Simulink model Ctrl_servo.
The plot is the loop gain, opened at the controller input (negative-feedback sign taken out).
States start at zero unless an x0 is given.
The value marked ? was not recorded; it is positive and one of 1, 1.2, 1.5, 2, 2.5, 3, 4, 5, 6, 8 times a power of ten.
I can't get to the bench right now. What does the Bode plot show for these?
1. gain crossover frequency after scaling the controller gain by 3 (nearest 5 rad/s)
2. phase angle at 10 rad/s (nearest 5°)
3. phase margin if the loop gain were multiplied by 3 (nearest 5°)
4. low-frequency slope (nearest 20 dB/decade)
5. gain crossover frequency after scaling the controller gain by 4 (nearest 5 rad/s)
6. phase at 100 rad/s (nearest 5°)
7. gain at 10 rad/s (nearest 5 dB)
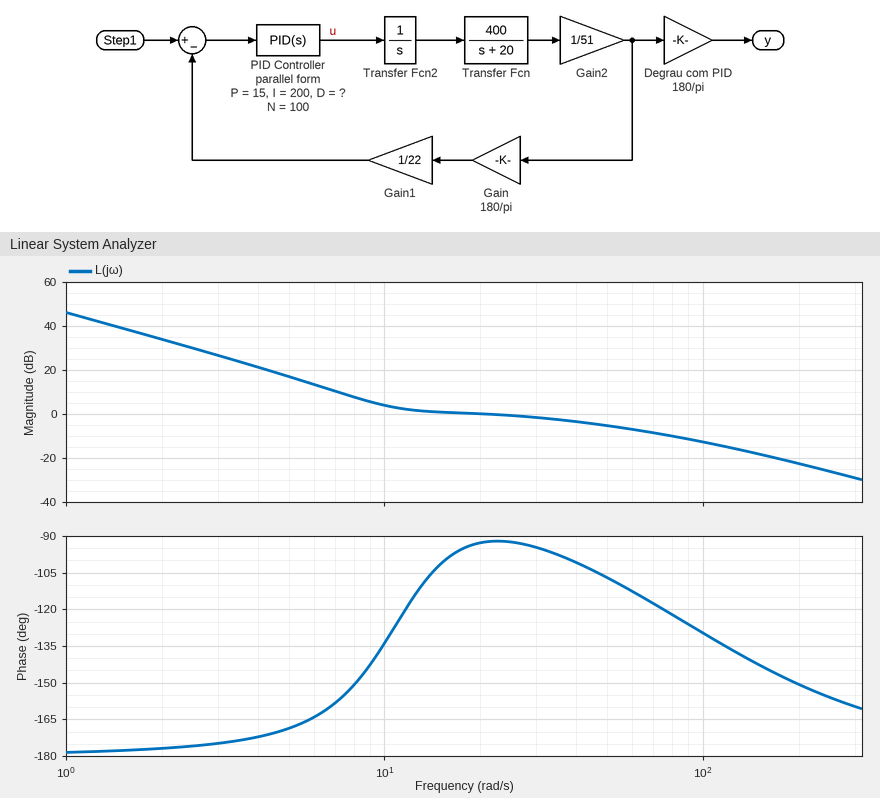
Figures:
75 rad/s
-135°
60°
-40 dB/decade
95 rad/s
-130°
5 dB
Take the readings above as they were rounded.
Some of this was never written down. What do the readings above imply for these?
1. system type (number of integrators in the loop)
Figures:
2
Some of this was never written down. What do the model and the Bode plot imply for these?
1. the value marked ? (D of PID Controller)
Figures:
1.5
